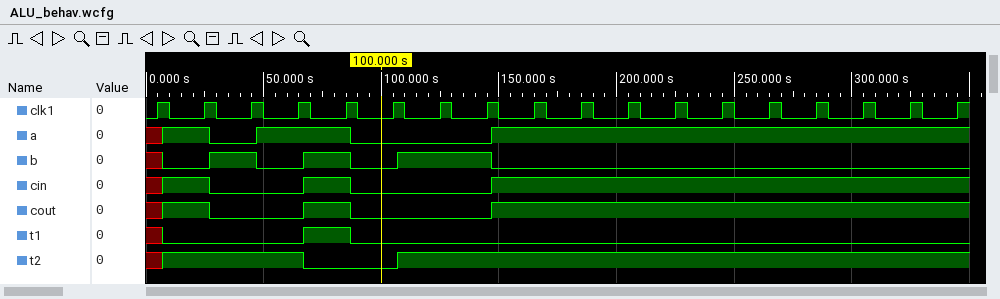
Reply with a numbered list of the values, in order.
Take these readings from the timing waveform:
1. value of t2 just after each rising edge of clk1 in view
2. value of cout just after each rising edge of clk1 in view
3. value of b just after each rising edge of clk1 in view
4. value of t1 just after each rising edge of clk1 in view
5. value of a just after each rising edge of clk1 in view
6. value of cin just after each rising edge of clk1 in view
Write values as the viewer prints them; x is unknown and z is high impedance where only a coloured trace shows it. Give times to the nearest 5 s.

1. x 1 1 1 0 0 1 1 1 1 1 1 1 1 1 1 1 1
2. x 1 0 0 1 0 0 0 1 1 1 1 1 1 1 1 1 1
3. x 0 1 0 1 0 1 1 0 0 0 0 0 0 0 0 0 0
4. x 0 0 0 1 0 0 0 0 0 0 0 0 0 0 0 0 0
5. x 1 0 1 1 0 0 0 1 1 1 1 1 1 1 1 1 1
6. x 1 0 0 1 0 0 0 1 1 1 1 1 1 1 1 1 1
